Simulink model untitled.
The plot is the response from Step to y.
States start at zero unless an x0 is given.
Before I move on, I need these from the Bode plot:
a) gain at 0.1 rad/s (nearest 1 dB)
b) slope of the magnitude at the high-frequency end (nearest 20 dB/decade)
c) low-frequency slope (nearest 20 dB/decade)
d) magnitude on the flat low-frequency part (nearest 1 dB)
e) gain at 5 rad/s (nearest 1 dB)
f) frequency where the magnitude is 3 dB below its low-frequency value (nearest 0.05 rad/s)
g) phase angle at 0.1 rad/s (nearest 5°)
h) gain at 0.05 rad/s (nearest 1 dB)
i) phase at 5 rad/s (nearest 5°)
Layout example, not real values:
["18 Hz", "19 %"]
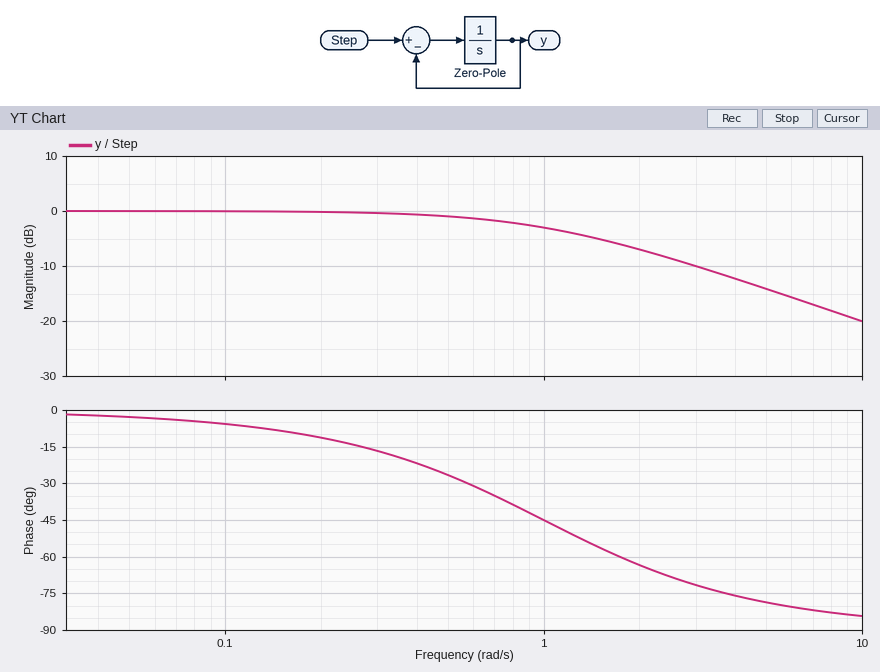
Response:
["0 dB", "-20 dB/decade", "0 dB/decade", "0 dB", "-14 dB", "1.00 rad/s", "-5°", "0 dB", "-80°"]
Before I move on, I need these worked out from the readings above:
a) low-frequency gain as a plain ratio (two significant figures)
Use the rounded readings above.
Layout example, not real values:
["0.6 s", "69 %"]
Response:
["1.0"]
